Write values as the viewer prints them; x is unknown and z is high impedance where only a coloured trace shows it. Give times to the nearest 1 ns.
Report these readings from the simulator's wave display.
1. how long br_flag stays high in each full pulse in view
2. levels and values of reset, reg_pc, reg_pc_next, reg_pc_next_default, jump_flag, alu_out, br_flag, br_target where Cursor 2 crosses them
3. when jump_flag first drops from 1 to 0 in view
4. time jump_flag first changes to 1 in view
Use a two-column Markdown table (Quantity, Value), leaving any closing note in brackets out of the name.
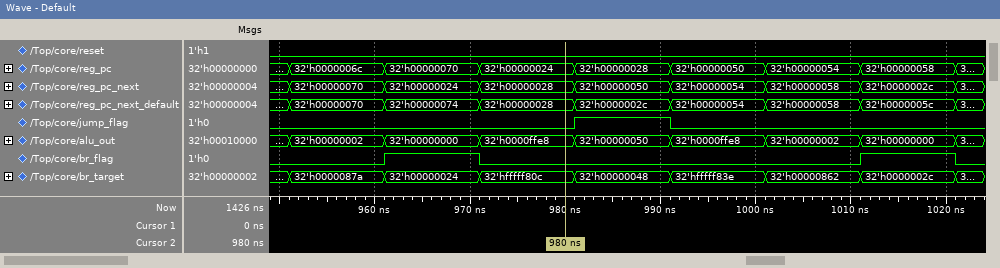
| Quantity | Value |
|---|---|
| how long br_flag stays high in each full pulse in view | 10 ns, 10 ns |
| levels and values of reset, reg_pc, reg_pc_next, reg_pc_next_default, jump_flag, alu_out, br_flag, br_target where Cursor 2 crosses them | reset=0, reg_pc=32'h00000024, reg_pc_next=32'h00000028, reg_pc_next_default=32'h00000028, jump_flag=0, alu_out=32'h0000ffe8, br_flag=0, br_target=32'hfffff80c |
| when jump_flag first drops from 1 to 0 in view | 991 ns |
| time jump_flag first changes to 1 in view | 981 ns |
